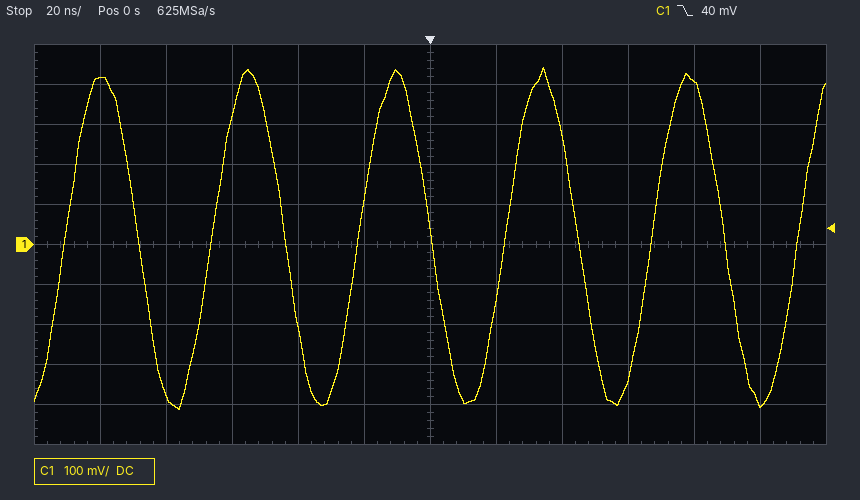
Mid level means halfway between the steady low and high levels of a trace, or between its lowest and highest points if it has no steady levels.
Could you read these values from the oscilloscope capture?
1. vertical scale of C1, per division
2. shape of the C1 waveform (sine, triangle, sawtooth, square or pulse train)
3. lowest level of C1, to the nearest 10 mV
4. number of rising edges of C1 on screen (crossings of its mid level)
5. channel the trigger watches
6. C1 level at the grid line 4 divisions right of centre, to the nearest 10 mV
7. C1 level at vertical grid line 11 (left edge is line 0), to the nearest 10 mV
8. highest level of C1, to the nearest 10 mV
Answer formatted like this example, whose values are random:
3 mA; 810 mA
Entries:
100 mV; sine; -410 mV; 6; C1; 410 mV; -400 mV; 440 mV
